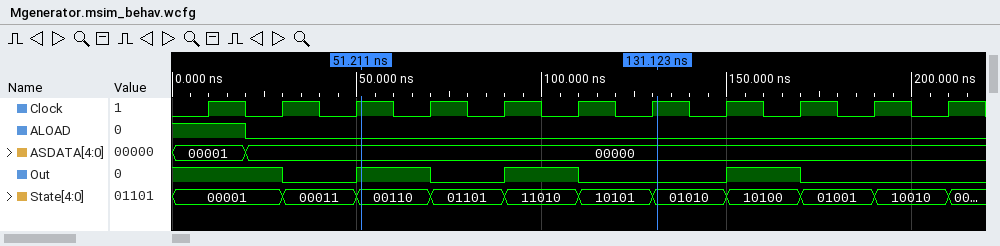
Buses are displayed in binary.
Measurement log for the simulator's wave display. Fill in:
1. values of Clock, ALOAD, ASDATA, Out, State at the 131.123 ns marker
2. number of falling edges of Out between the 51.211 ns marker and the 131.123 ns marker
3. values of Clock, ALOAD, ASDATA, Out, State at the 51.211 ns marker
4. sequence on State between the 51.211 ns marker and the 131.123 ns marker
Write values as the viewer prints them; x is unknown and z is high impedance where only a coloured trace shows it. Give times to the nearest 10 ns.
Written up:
Clock=1, ALOAD=0, ASDATA=00000, Out=0, State=01010
2
Clock=1, ALOAD=0, ASDATA=00000, Out=1, State=00110
00110, 01101, 11010, 10101, 01010
